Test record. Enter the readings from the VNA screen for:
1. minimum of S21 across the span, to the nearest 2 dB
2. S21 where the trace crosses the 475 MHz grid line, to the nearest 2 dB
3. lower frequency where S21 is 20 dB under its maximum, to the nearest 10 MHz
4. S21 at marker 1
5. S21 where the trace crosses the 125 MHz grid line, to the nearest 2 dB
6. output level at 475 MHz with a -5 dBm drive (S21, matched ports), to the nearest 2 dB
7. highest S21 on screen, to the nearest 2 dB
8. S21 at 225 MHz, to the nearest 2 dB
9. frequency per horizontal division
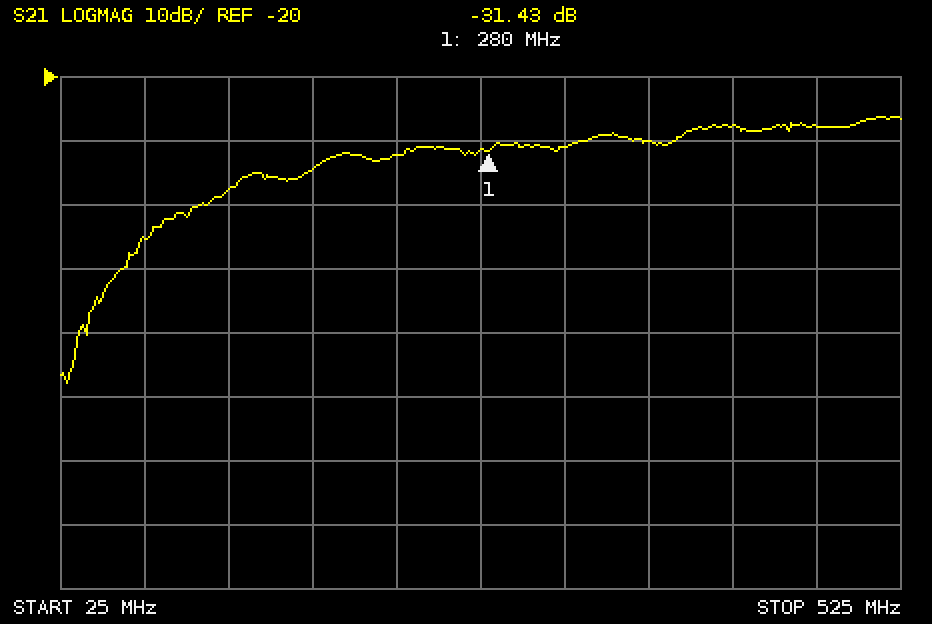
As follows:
-68 dB
-28 dB
70 MHz
-31.43 dB
-38 dB
-32 dBm
-26 dB
-32 dB
50 MHz
